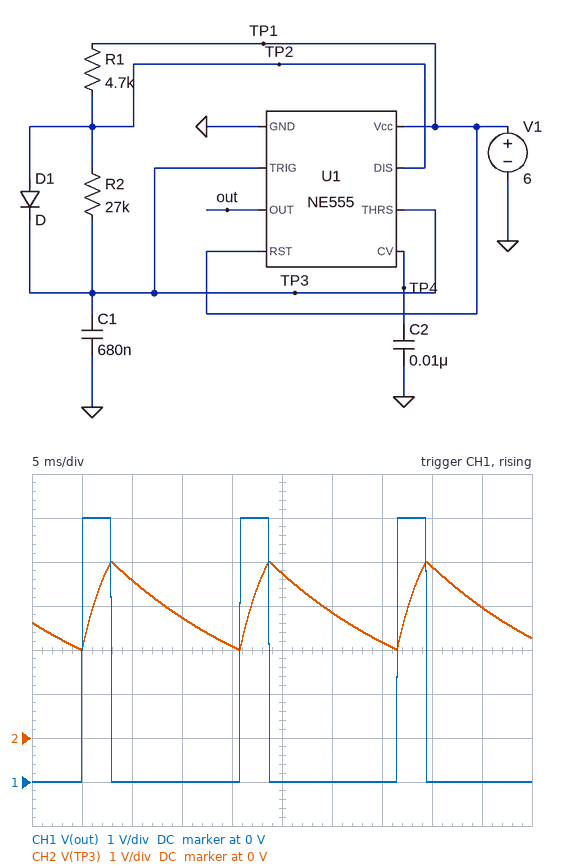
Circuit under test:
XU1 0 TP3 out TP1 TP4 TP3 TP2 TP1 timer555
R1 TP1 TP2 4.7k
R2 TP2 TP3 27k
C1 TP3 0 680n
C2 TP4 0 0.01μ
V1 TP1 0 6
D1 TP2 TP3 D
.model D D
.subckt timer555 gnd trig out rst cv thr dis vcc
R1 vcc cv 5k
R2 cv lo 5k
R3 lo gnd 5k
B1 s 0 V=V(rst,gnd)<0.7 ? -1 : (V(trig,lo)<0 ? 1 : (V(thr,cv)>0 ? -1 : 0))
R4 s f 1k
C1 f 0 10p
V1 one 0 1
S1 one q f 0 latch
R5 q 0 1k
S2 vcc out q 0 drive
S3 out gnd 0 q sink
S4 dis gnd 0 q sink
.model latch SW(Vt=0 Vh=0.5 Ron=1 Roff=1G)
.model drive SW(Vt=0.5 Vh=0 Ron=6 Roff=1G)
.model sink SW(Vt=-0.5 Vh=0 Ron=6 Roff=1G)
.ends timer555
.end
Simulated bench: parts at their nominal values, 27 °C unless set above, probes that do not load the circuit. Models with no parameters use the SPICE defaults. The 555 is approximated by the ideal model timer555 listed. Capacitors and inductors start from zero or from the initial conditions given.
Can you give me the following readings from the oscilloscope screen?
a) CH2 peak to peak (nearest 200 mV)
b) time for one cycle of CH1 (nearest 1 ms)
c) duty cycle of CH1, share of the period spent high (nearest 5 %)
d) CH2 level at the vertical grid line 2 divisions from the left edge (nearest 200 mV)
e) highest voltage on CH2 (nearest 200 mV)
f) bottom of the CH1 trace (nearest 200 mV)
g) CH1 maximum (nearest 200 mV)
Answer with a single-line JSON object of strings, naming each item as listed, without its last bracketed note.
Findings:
{"CH2 peak to peak": "2.0 V", "time for one cycle of CH1": "16 ms", "duty cycle of CH1, share of the period spent high": "20 %", "CH2 level at the vertical grid line 2 divisions from the left edge": "3.6 V", "highest voltage on CH2": "4.0 V", "bottom of the CH1 trace": "0 V", "CH1 maximum": "6.0 V"}
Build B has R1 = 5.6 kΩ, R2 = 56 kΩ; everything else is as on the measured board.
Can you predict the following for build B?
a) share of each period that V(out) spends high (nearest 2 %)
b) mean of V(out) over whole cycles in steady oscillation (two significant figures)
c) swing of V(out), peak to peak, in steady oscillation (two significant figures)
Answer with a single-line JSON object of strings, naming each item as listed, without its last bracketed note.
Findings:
{"share of each period that V(out) spends high": "12 %", "mean of V(out) over whole cycles in steady oscillation": "690 mV", "swing of V(out), peak to peak, in steady oscillation": "6.0 V"}
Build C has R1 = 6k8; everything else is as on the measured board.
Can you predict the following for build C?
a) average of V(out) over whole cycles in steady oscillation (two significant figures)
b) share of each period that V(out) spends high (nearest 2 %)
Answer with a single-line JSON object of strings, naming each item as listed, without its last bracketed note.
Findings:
{"average of V(out) over whole cycles in steady oscillation": "1.5 V", "share of each period that V(out) spends high": "24 %"}
